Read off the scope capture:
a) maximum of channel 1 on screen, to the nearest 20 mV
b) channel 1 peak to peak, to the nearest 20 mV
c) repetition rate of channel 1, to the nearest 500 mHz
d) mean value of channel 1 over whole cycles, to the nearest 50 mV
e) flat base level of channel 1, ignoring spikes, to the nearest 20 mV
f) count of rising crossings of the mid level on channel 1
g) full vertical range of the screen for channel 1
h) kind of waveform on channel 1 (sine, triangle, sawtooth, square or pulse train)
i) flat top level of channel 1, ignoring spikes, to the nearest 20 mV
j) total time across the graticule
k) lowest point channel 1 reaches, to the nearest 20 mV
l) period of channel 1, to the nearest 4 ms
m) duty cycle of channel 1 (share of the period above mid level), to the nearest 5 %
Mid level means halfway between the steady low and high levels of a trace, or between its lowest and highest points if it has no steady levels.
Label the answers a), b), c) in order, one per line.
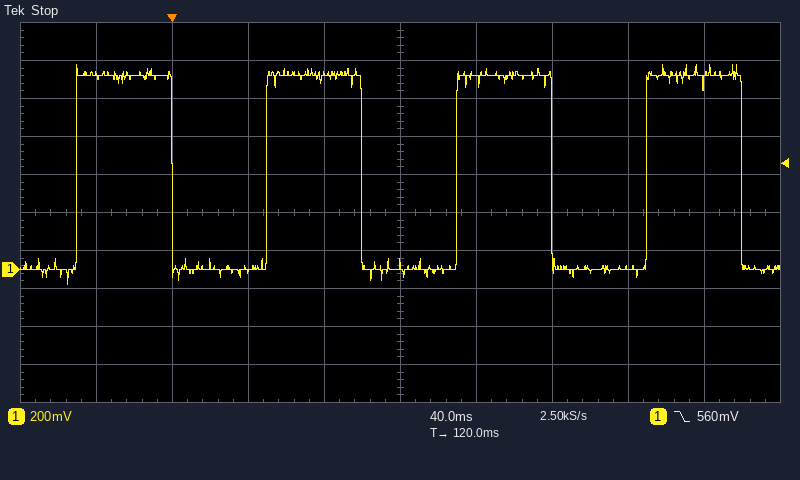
a) 1.08 V
b) 1.16 V
c) 10.0 Hz
d) 500 mV
e) 0 mV
f) 4
g) 2 V
h) square
i) 1.02 V
j) 400 ms
k) -80 mV
l) 100 ms
m) 50 %
